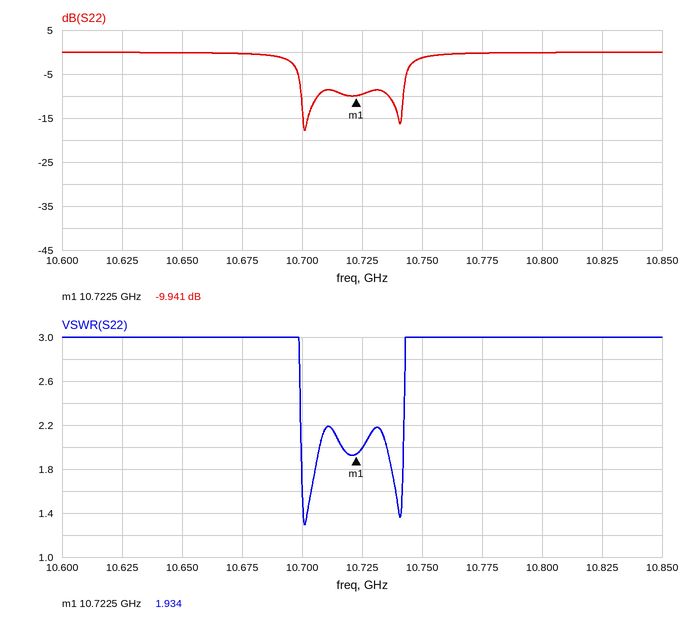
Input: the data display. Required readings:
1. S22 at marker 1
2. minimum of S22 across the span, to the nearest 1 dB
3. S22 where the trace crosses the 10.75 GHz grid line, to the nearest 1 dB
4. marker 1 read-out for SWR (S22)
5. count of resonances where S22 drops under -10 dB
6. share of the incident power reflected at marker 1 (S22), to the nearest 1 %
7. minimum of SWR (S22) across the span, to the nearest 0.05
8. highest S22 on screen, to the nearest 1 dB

-9.941 dB
-18 dB
-1 dB
1.934
2
10 %
1.30
0 dB
